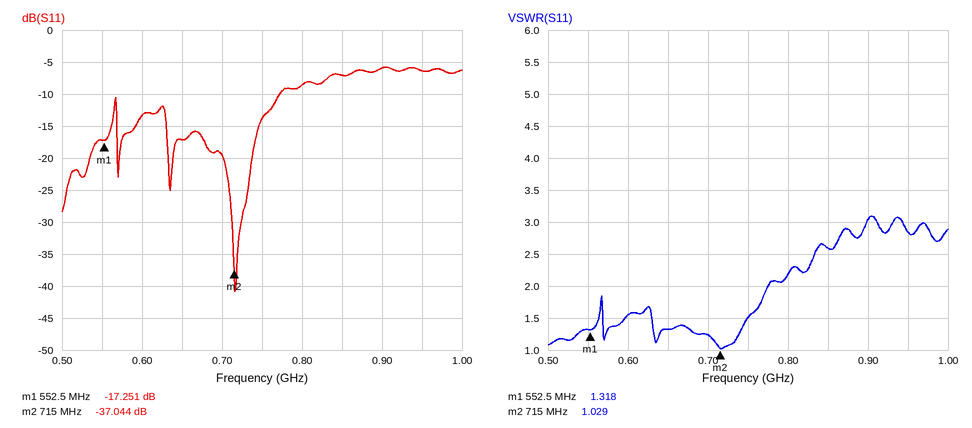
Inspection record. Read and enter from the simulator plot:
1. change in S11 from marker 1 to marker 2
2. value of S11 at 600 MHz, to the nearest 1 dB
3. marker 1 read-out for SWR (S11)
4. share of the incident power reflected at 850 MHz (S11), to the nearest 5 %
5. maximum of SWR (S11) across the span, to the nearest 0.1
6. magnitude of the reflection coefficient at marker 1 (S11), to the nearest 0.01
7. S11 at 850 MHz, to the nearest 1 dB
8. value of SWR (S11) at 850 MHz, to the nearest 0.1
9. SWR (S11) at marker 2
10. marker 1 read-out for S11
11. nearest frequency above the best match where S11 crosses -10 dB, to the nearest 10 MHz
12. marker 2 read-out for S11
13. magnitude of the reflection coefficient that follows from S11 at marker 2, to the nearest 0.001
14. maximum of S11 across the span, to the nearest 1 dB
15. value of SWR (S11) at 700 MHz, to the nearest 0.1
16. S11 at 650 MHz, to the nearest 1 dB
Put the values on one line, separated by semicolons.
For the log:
-19.793 dB; -13 dB; 1.318; 20 %; 3.1; 0.14; -7 dB; 2.6; 1.029; -17.251 dB; 770 MHz; -37.044 dB; 0.014; -6 dB; 1.2; -17 dB
